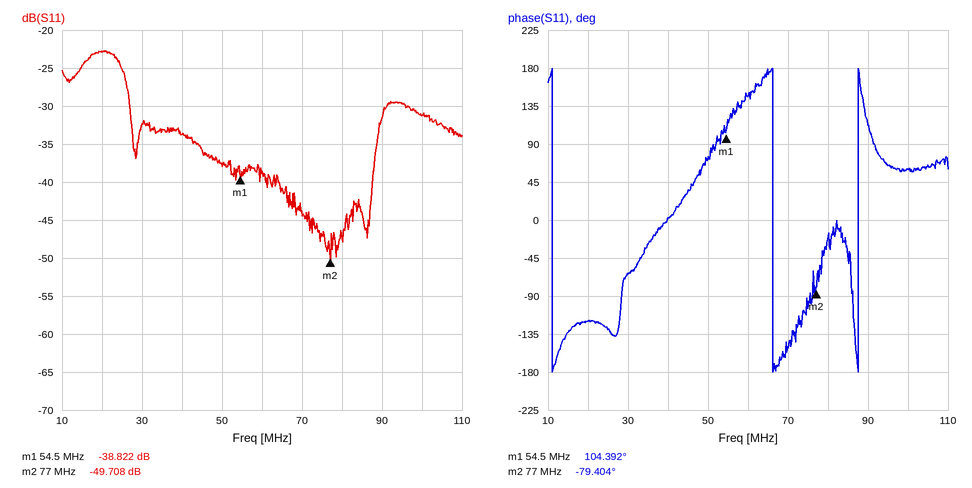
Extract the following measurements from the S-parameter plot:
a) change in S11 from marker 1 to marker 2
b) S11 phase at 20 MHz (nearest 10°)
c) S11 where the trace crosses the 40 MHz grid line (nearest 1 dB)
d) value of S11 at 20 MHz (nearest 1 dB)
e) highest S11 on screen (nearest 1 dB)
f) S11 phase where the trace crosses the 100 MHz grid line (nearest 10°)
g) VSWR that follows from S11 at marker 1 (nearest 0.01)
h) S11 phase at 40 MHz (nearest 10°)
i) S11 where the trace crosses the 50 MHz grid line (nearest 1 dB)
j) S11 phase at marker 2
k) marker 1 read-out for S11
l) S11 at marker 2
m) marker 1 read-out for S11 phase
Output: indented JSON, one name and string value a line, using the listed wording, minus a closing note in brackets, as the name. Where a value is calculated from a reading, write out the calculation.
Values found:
{
  "change in S11 from marker 1 to marker 2": "-49.708 − (-38.822) = -10.886 dB",
  "S11 phase at 20 MHz": "-120°",
  "S11 where the trace crosses the 40 MHz grid line": "-34 dB",
  "value of S11 at 20 MHz": "-23 dB",
  "highest S11 on screen": "-23 dB",
  "S11 phase where the trace crosses the 100 MHz grid line": "60°",
  "VSWR that follows from S11 at marker 1": "(1 + 0.0115)/(1 − 0.0115) ≈ 1.02",
  "S11 phase at 40 MHz": "0°",
  "S11 where the trace crosses the 50 MHz grid line": "-38 dB",
  "S11 phase at marker 2": "-79.404°",
  "marker 1 read-out for S11": "-38.822 dB",
  "S11 at marker 2": "-49.708 dB",
  "marker 1 read-out for S11 phase": "104.392°"
}
